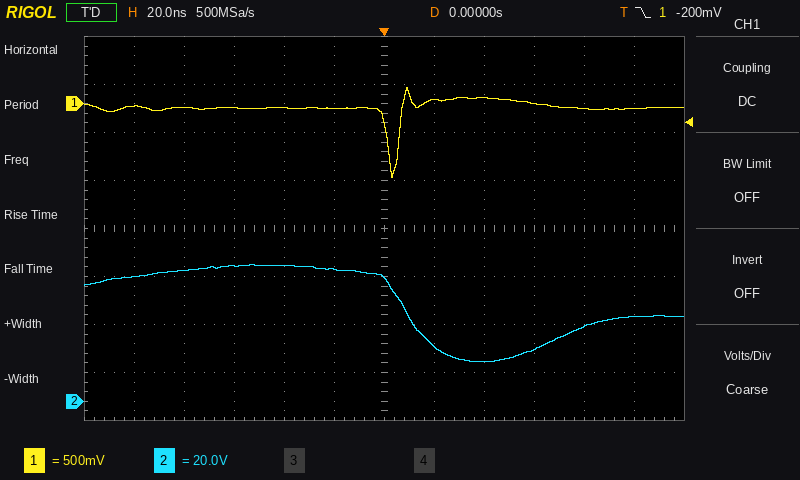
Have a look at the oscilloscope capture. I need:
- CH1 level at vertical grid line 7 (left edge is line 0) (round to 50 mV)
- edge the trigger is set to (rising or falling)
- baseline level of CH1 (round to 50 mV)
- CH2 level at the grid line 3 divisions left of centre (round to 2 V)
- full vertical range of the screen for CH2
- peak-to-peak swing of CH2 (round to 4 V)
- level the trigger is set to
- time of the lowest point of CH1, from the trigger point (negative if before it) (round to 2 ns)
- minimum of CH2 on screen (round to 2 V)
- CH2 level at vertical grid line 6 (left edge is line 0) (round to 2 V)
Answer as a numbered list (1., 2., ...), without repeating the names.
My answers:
1. 50 mV
2. falling
3. -50 mV
4. 56 V
5. 160 V
6. 40 V
7. -200 mV
8. +4 ns
9. 16 V
10. 52 V
